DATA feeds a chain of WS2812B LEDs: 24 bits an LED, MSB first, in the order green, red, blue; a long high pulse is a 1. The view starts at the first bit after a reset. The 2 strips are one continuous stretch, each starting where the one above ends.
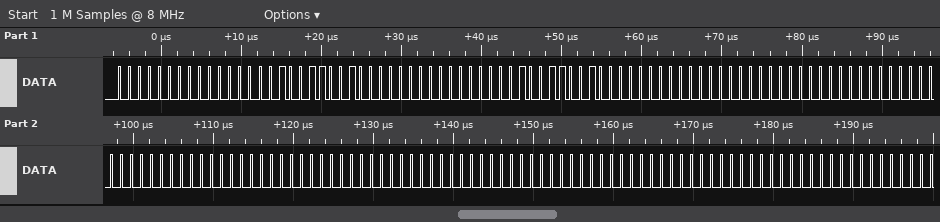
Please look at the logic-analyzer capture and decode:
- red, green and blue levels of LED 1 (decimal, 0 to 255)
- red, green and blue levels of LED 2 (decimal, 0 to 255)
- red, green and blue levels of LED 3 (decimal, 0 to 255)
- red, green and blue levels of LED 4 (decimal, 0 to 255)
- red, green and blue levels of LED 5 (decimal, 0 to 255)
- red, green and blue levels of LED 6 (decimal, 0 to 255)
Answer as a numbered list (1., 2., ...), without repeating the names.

1. 0, 0, 153
2. 0, 0, 153
3. 0, 0, 0
4. 0, 0, 0
5. 0, 0, 0
6. 0, 0, 0
